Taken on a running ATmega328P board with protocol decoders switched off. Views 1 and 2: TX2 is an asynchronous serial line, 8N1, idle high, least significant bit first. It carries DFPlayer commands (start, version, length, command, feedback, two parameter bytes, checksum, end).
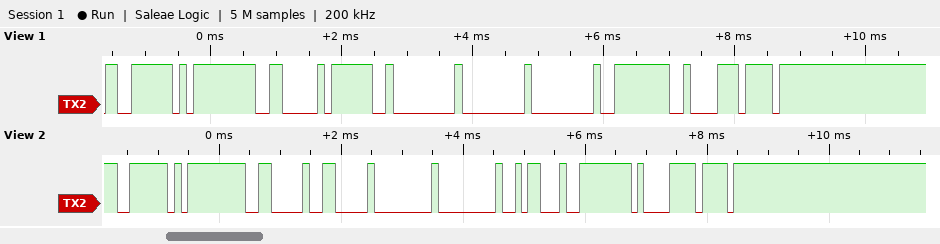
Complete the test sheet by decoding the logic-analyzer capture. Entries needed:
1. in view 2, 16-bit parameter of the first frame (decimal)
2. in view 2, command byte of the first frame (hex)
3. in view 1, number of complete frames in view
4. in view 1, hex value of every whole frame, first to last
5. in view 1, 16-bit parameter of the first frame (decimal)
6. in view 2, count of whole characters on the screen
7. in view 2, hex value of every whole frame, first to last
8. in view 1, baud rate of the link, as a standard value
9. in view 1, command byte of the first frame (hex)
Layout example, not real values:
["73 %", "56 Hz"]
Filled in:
["26", "0x06", "10", "7E FF 06 3F 00 00 00 FE C2 EF", "0", "10", "7E FF 06 06 00 00 1A FE E1 EF", "9600 baud", "0x3F"]
